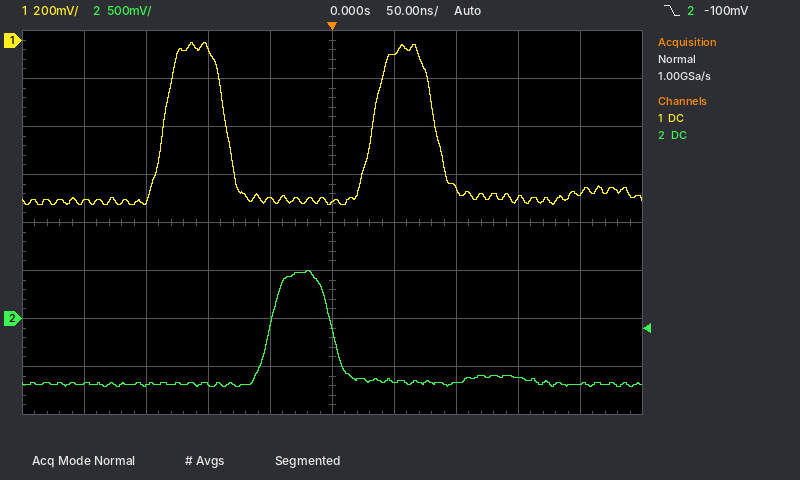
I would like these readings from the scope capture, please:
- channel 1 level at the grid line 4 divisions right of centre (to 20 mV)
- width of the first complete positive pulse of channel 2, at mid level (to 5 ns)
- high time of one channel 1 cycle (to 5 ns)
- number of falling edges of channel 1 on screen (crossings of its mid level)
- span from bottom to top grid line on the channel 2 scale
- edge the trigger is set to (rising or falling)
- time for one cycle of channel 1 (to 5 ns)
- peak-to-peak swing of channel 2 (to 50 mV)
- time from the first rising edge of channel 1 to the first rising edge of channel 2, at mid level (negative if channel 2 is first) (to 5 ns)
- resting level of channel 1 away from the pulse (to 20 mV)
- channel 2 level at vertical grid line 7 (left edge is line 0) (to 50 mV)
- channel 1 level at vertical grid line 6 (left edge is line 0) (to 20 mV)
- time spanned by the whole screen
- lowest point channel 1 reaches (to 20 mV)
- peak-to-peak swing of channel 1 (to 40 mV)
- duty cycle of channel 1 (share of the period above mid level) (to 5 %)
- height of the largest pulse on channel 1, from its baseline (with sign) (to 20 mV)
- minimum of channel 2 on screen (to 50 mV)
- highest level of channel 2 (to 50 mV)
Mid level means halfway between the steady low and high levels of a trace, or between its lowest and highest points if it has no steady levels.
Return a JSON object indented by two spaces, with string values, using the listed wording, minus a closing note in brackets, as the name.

{
  "channel 1 level at the grid line 4 divisions right of centre": "-640 mV",
  "width of the first complete positive pulse of channel 2, at mid level": "50 ns",
  "high time of one channel 1 cycle": "50 ns",
  "number of falling edges of channel 1 on screen": "2",
  "span from bottom to top grid line on the channel 2 scale": "4 V",
  "edge the trigger is set to": "falling",
  "time for one cycle of channel 1": "170 ns",
  "peak-to-peak swing of channel 2": "1.20 V",
  "time from the first rising edge of channel 1 to the first rising edge of channel 2, at mid level (negative if channel 2 is first)": "+85 ns",
  "resting level of channel 1 away from the pulse": "-660 mV",
  "channel 2 level at vertical grid line 7 (left edge is line 0)": "-650 mV",
  "channel 1 level at vertical grid line 6 (left edge is line 0)": "-60 mV",
  "time spanned by the whole screen": "500 ns",
  "lowest point channel 1 reaches": "-680 mV",
  "peak-to-peak swing of channel 1": "680 mV",
  "duty cycle of channel 1 (share of the period above mid level)": "30 %",
  "height of the largest pulse on channel 1, from its baseline (with sign)": "+640 mV",
  "minimum of channel 2 on screen": "-700 mV",
  "highest level of channel 2": "500 mV"
}
